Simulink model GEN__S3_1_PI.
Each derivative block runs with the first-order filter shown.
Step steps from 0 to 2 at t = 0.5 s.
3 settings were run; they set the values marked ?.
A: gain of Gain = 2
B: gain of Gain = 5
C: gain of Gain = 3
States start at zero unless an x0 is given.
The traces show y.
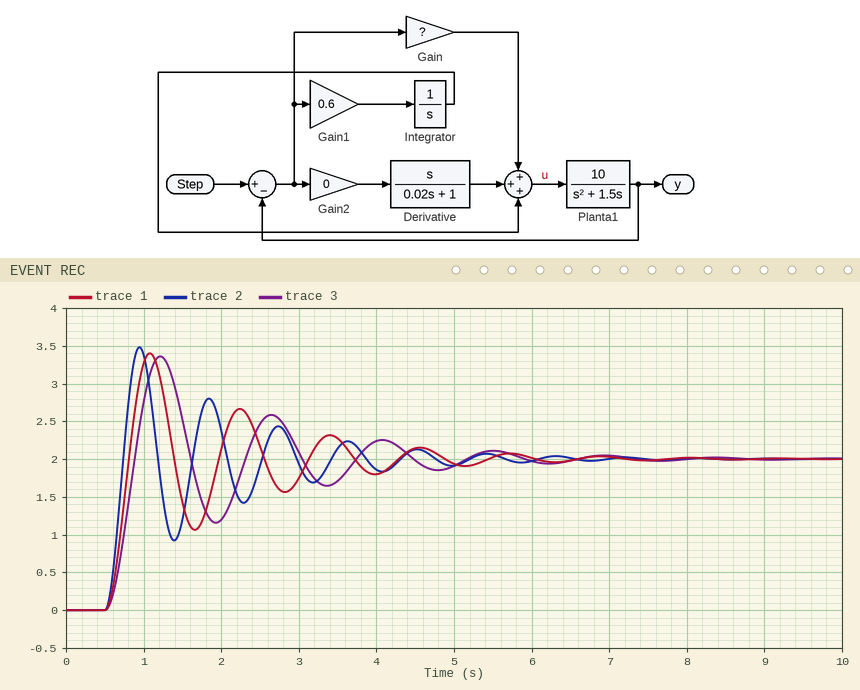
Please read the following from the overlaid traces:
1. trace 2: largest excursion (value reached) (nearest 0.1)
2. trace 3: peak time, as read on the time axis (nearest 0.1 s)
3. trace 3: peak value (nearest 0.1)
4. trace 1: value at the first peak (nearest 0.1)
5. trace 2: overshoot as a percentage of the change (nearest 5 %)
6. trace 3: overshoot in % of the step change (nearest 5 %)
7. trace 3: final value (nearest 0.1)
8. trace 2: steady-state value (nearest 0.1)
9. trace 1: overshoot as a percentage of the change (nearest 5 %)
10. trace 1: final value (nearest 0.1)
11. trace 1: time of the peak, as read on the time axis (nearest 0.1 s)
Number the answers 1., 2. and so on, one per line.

1. 3.5
2. 1.2 s
3. 3.4
4. 3.4
5. 75 %
6. 70 %
7. 2.0
8. 2.0
9. 70 %
10. 2.0
11. 1.1 s
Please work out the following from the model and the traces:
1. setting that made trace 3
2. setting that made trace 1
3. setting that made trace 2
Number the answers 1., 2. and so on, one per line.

1. A
2. C
3. B
